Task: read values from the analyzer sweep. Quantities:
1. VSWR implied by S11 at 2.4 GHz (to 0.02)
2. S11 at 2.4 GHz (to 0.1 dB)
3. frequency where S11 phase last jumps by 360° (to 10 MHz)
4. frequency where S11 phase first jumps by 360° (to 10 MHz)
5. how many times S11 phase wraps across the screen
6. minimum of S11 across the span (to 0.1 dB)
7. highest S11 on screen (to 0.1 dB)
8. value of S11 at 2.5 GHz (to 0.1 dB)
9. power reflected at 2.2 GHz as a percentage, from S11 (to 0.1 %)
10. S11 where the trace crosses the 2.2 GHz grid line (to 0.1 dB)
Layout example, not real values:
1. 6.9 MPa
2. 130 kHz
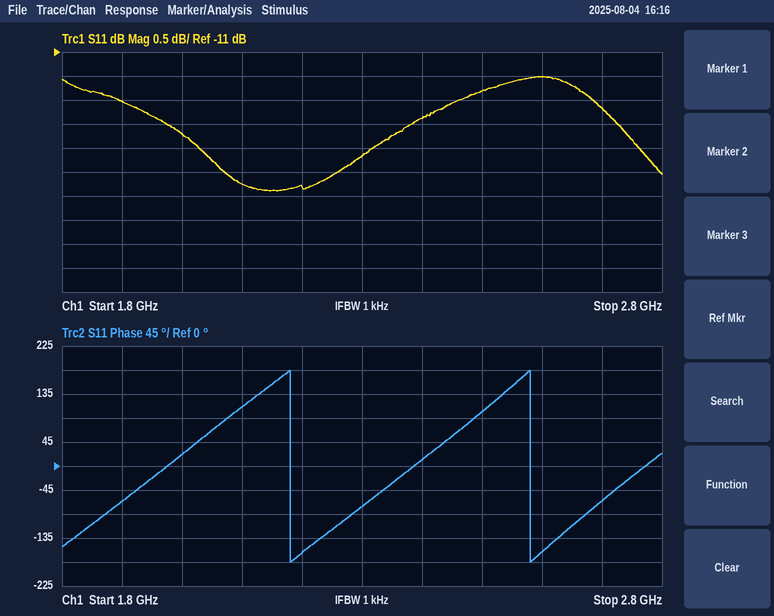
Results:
1. 1.64
2. -12.4 dB
3. 2.58 GHz
4. 2.18 GHz
5. 2
6. -13.9 dB
7. -11.5 dB
8. -11.8 dB
9. 4.2 %
10. -13.8 dB
